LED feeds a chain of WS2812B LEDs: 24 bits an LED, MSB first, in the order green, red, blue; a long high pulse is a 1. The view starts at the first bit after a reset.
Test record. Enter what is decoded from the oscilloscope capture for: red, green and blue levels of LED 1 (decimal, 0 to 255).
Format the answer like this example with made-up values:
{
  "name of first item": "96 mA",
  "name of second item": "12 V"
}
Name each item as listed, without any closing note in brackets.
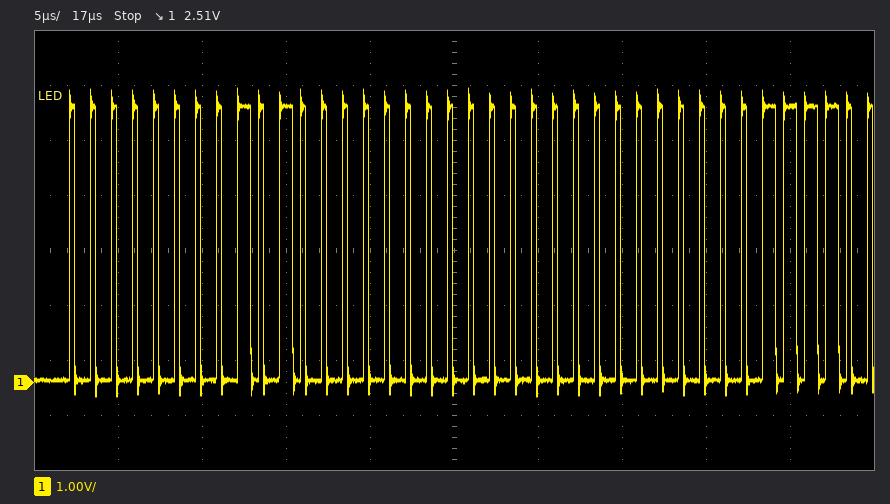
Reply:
{
  "red, green and blue levels of LED 1": "160, 0, 0"
}
